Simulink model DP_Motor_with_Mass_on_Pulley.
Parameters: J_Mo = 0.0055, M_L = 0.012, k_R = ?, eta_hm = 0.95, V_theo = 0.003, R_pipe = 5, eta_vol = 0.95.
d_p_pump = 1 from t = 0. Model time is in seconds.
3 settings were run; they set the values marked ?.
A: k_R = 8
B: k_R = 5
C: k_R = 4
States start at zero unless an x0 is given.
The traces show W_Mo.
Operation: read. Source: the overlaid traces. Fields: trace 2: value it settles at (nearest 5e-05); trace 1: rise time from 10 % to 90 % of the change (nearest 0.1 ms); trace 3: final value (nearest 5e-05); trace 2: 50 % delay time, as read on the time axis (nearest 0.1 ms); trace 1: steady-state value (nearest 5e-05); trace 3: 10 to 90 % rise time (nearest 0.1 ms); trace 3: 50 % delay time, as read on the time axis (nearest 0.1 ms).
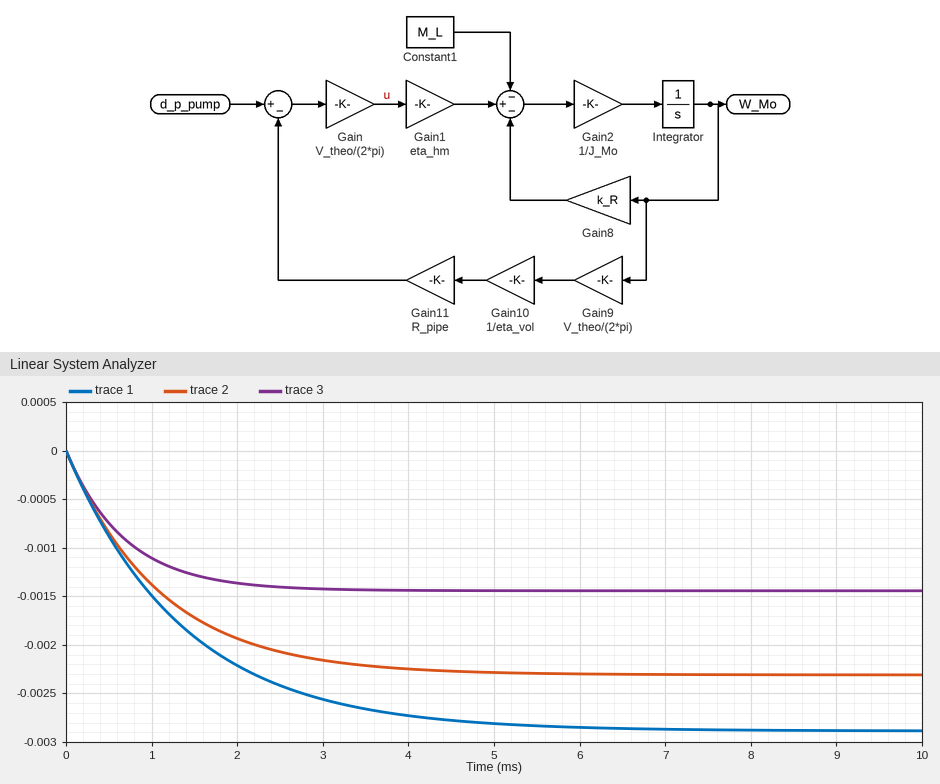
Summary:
-0.00230
3.0 ms
-0.00145
0.8 ms
-0.00290
1.5 ms
0.5 ms
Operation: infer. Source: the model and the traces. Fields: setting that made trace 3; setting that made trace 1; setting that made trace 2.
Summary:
A
C
B
